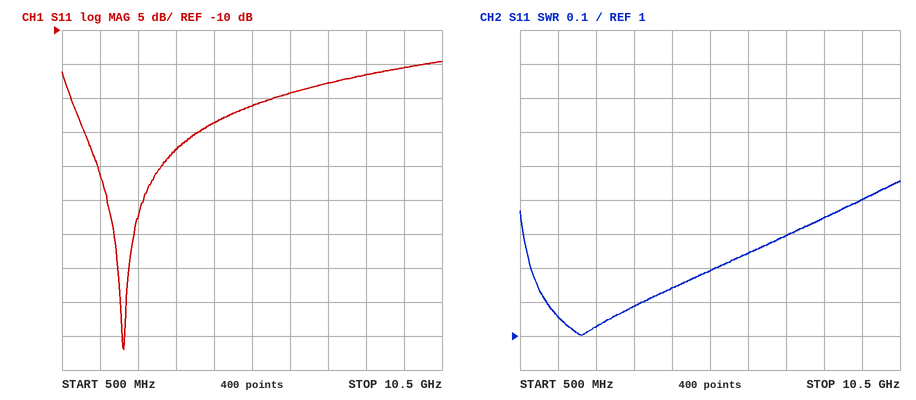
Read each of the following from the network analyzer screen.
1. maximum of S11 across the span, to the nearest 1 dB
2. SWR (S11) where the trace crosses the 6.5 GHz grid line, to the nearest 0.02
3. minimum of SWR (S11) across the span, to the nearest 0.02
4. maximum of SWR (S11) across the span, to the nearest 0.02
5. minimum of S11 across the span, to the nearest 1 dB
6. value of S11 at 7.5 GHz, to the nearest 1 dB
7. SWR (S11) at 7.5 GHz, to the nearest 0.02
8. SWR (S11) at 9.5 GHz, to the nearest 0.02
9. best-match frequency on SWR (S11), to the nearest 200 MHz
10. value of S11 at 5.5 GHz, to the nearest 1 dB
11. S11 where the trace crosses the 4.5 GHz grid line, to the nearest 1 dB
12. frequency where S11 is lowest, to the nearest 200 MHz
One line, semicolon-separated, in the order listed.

-15 dB; 1.24; 1.00; 1.46; -57 dB; -18 dB; 1.30; 1.40; 2.2 GHz; -21 dB; -24 dB; 2.2 GHz
